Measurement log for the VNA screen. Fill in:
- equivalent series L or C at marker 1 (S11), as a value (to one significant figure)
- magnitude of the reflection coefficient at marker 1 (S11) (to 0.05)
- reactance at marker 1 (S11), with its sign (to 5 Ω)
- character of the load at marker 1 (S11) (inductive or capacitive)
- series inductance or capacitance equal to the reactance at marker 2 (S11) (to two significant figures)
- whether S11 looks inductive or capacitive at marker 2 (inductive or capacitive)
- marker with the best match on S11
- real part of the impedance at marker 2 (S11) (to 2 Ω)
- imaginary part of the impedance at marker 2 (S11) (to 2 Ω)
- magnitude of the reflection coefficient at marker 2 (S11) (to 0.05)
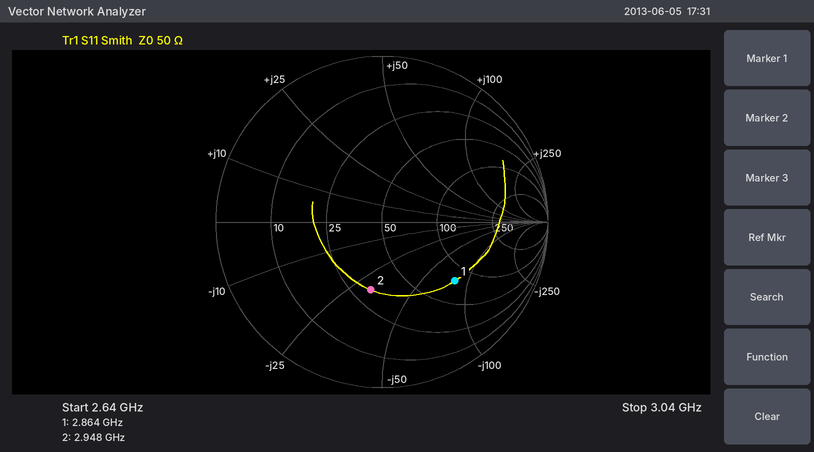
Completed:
700 fF
0.55
-80 Ω
capacitive
1.7 pF
capacitive
marker 2
32 Ω
-32 Ω
0.40
